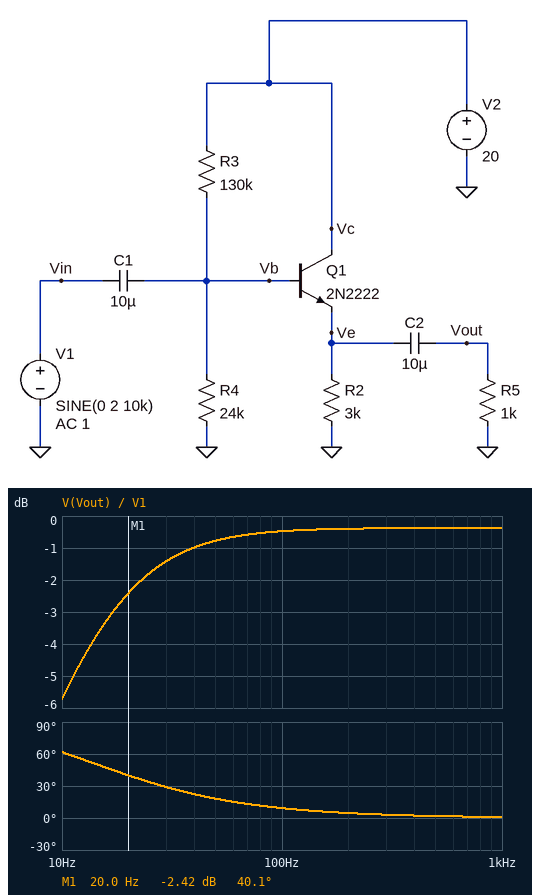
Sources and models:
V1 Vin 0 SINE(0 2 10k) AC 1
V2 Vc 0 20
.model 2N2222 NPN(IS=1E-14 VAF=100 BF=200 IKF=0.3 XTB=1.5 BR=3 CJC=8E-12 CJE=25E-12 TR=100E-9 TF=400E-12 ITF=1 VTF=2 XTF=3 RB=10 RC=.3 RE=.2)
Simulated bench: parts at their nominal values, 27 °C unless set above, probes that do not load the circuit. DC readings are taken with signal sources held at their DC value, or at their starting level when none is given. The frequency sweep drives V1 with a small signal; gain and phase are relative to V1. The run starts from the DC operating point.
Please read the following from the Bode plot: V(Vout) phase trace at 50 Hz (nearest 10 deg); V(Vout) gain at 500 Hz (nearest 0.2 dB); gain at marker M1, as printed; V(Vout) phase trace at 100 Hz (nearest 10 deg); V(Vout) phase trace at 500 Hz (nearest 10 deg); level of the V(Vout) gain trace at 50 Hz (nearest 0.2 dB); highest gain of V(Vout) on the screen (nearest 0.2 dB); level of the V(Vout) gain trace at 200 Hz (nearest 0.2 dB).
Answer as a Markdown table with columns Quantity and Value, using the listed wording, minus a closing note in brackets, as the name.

| Quantity | Value |
|---|---|
| V(Vout) phase trace at 50 Hz | 20 deg |
| V(Vout) gain at 500 Hz | -0.4 dB |
| gain at marker M1, as printed | -2.42 dB |
| V(Vout) phase trace at 100 Hz | 10 deg |
| V(Vout) phase trace at 500 Hz | 0 deg |
| level of the V(Vout) gain trace at 50 Hz | -0.8 dB |
| highest gain of V(Vout) on the screen | -0.4 dB |
| level of the V(Vout) gain trace at 200 Hz | -0.4 dB |
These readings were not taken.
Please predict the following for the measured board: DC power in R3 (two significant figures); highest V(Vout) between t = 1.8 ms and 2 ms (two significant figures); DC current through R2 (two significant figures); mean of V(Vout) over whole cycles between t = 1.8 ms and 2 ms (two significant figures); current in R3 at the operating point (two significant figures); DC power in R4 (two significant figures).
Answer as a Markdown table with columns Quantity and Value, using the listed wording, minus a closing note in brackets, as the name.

| Quantity | Value |
|---|---|
| DC power in R3 | 2.2 mW |
| highest V(Vout) between t = 1.8 ms and 2 ms | 1.9 V |
| DC current through R2 | 800 µA |
| mean of V(Vout) over whole cycles between t = 1.8 ms and 2 ms | 310 mV |
| current in R3 at the operating point | 130 µA |
| DC power in R4 | 390 µW |
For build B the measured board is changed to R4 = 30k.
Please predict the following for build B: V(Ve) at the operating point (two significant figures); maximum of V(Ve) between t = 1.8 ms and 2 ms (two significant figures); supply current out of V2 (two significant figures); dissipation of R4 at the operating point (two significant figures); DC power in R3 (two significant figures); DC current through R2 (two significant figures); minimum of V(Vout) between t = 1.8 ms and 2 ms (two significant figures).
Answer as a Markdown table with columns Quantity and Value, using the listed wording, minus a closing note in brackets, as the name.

| Quantity | Value |
|---|---|
| V(Ve) at the operating point | 3.0 V |
| maximum of V(Ve) between t = 1.8 ms and 2 ms | 5.0 V |
| supply current out of V2 | 1.1 mA |
| dissipation of R4 at the operating point | 440 µW |
| DC power in R3 | 2.1 mW |
| DC current through R2 | 1.0 mA |
| minimum of V(Vout) between t = 1.8 ms and 2 ms | -770 mV |
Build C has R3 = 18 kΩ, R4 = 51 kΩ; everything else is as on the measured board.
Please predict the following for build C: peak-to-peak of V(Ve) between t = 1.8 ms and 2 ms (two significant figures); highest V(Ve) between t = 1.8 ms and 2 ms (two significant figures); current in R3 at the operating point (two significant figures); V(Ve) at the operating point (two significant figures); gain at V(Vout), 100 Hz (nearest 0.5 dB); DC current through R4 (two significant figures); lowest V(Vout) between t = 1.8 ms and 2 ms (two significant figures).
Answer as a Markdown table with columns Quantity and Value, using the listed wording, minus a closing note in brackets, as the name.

| Quantity | Value |
|---|---|
| peak-to-peak of V(Ve) between t = 1.8 ms and 2 ms | 4.0 V |
| highest V(Ve) between t = 1.8 ms and 2 ms | 16 V |
| current in R3 at the operating point | 310 µA |
| V(Ve) at the operating point | 14 V |
| gain at V(Vout), 100 Hz | 0 dB |
| DC current through R4 | 280 µA |
| lowest V(Vout) between t = 1.8 ms and 2 ms | -2.0 V |
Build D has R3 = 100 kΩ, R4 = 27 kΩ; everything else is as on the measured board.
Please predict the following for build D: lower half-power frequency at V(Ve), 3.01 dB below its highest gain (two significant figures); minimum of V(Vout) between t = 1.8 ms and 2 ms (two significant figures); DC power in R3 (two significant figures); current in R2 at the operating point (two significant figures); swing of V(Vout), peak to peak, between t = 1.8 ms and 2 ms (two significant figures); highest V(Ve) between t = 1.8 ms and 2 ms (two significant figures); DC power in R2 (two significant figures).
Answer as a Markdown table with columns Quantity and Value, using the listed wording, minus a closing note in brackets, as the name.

| Quantity | Value |
|---|---|
| lower half-power frequency at V(Ve), 3.01 dB below its highest gain | 760 mHz |
| minimum of V(Vout) between t = 1.8 ms and 2 ms | -890 mV |
| DC power in R3 | 2.5 mW |
| current in R2 at the operating point | 1.2 mA |
| swing of V(Vout), peak to peak, between t = 1.8 ms and 2 ms | 2.8 V |
| highest V(Ve) between t = 1.8 ms and 2 ms | 5.5 V |
| DC power in R2 | 4.1 mW |
